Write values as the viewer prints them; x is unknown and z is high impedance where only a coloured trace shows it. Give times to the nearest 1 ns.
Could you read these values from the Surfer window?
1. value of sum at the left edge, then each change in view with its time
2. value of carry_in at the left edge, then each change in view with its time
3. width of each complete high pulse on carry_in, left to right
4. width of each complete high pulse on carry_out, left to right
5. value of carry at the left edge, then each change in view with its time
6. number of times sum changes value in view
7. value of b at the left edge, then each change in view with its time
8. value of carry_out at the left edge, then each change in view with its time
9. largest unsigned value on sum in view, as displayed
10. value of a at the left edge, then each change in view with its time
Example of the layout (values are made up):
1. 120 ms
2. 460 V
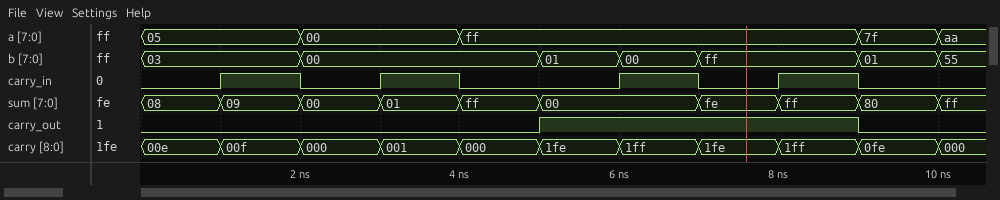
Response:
1. 08, 09 at 1 ns, 00 at 2 ns, 01 at 3 ns, ff at 4 ns, 00 at 5 ns, fe at 7 ns, ff at 8 ns, 80 at 9 ns, ff at 10 ns
2. 0, 1 at 1 ns, 0 at 2 ns, 1 at 3 ns, 0 at 4 ns, 1 at 6 ns, 0 at 7 ns, 1 at 8 ns, 0 at 9 ns
3. 1 ns, 1 ns, 1 ns, 1 ns
4. 4 ns
5. 00e, 00f at 1 ns, 000 at 2 ns, 001 at 3 ns, 000 at 4 ns, 1fe at 5 ns, 1ff at 6 ns, 1fe at 7 ns, 1ff at 8 ns, 0fe at 9 ns, 000 at 10 ns
6. 9
7. 03, 00 at 2 ns, 01 at 5 ns, 00 at 6 ns, ff at 7 ns, 01 at 9 ns, 55 at 10 ns
8. 0, 1 at 5 ns, 0 at 9 ns
9. ff
10. 05, 00 at 2 ns, ff at 4 ns, 7f at 9 ns, aa at 10 ns
